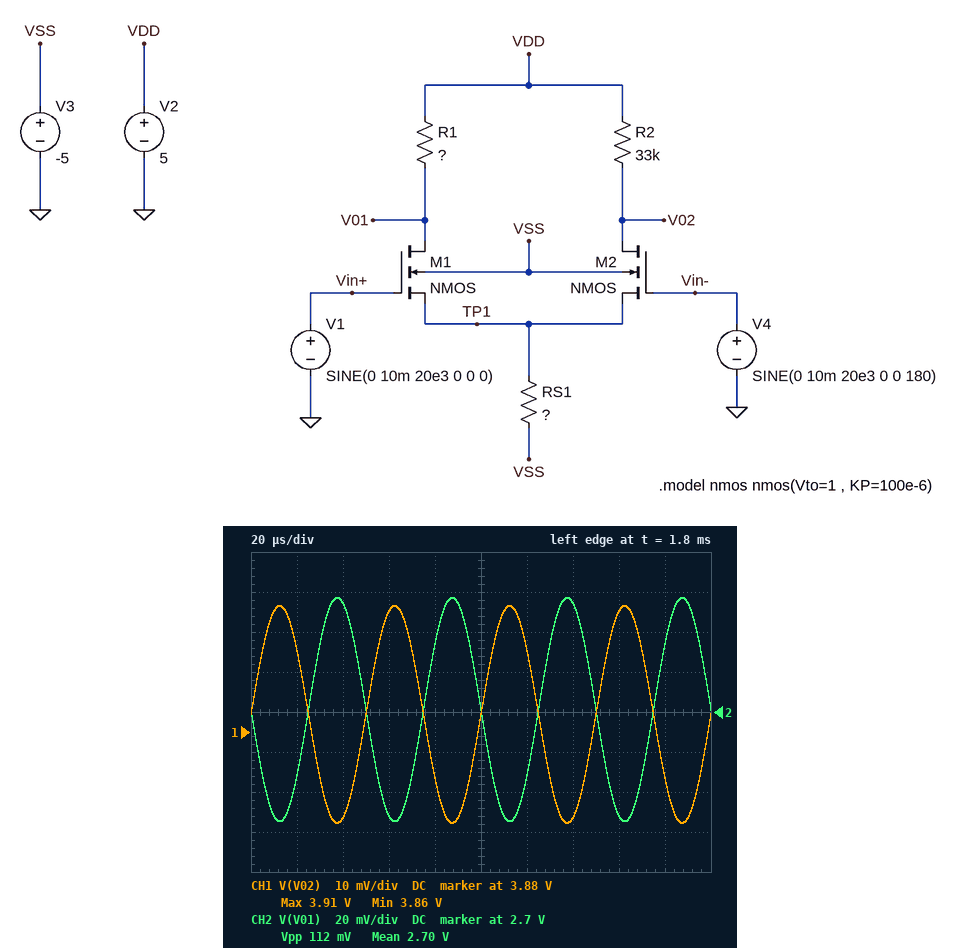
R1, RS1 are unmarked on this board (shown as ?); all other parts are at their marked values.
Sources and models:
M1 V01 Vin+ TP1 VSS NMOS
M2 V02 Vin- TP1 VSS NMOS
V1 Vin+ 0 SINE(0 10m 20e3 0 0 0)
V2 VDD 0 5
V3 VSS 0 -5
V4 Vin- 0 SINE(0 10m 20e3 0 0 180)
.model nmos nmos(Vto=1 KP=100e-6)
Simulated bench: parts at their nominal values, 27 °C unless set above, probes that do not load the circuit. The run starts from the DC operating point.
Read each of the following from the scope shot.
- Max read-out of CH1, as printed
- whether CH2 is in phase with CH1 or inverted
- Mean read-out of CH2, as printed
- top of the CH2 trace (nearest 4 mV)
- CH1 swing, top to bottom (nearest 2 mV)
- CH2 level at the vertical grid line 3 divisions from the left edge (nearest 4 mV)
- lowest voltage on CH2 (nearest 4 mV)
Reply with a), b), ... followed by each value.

a) 3.91 V
b) inverted
c) 2.70 V
d) 2.756 V
e) 54 mV
f) 2.648 V
g) 2.644 V
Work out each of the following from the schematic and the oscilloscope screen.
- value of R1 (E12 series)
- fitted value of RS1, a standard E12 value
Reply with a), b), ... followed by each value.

a) 68 kΩ
b) 47 kΩ
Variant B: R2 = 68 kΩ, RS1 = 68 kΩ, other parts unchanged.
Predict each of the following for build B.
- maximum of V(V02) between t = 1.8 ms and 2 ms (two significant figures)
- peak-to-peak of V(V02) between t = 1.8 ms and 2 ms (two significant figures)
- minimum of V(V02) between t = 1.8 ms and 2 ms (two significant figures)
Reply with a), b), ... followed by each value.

a) 3.4 V
b) 95 mV
c) 3.3 V
